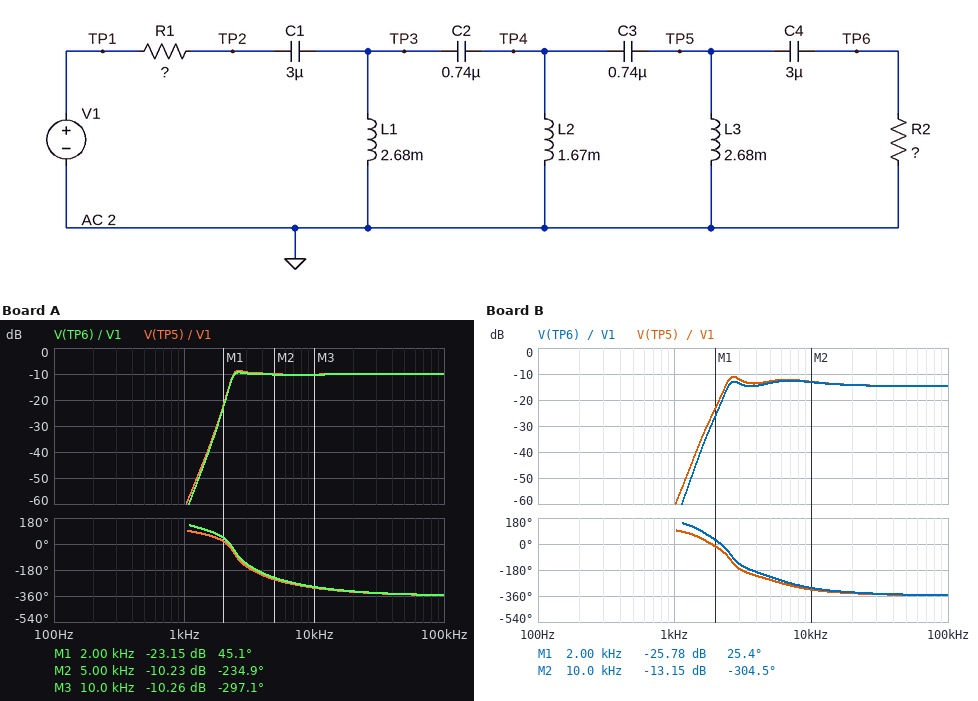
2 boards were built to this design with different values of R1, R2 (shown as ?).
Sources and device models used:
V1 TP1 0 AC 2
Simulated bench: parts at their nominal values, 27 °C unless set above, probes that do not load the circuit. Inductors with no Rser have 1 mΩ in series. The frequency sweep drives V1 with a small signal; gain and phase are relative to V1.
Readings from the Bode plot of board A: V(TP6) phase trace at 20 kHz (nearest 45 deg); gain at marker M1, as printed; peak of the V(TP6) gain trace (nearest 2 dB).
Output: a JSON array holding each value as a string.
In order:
["-315 deg", "-23.15 dB", "-10 dB"]
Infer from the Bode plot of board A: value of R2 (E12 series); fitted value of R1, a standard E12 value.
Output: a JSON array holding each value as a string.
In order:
["56 Ω", "120 Ω"]
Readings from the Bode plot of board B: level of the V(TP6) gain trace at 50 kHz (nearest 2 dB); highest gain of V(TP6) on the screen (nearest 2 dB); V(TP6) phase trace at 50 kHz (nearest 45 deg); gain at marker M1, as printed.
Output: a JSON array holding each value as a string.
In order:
["-14 dB", "-12 dB", "-360 deg", "-25.78 dB"]
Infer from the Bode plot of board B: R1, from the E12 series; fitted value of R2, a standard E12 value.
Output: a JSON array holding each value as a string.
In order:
["120 Ω", "27 Ω"]
